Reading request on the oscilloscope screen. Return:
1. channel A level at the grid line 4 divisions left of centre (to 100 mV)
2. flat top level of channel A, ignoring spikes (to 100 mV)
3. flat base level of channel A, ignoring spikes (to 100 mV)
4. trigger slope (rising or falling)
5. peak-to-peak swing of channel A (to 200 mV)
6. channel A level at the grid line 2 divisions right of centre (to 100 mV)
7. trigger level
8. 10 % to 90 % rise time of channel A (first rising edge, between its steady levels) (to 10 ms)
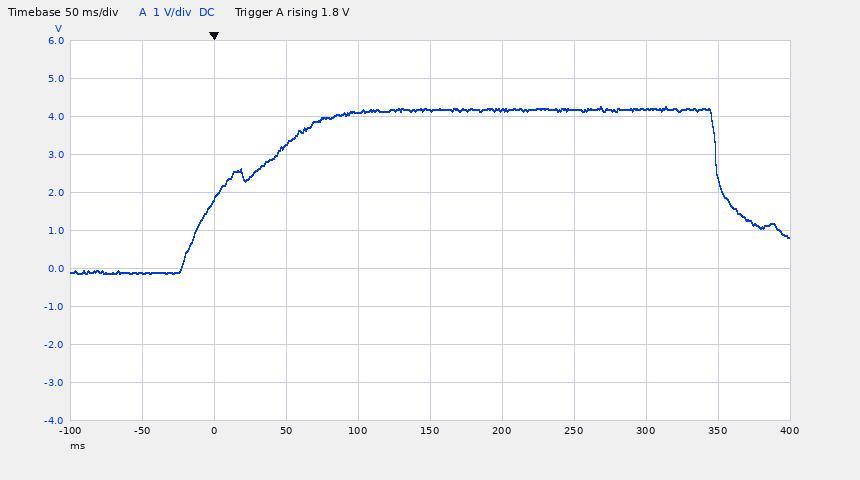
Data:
-100 mV
4.2 V
-100 mV
rising
4.4 V
4.2 V
1.8 V
90 ms
